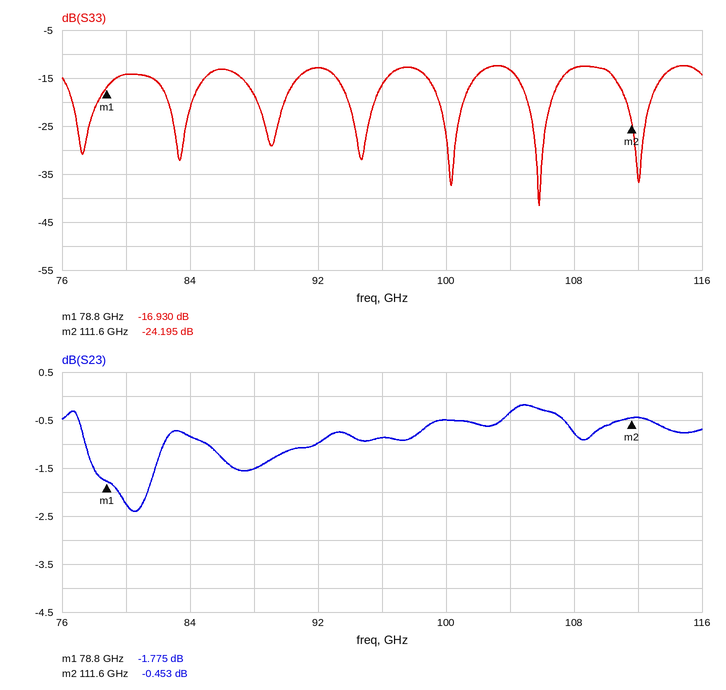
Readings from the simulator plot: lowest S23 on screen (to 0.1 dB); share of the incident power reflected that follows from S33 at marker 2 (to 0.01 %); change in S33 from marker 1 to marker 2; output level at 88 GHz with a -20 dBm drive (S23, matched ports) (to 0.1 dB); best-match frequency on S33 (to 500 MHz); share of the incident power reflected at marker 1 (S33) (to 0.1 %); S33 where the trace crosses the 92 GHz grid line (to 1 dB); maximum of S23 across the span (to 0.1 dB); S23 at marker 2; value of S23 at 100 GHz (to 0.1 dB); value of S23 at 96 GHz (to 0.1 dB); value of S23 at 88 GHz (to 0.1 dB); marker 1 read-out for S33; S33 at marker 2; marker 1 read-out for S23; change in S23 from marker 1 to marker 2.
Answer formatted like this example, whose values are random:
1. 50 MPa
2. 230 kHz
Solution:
1. -2.4 dB
2. 0.38 %
3. -7.265 dB
4. -21.5 dBm
5. 106.0 GHz
6. 2.0 %
7. -13 dB
8. -0.2 dB
9. -0.453 dB
10. -0.5 dB
11. -0.9 dB
12. -1.5 dB
13. -16.930 dB
14. -24.195 dB
15. -1.775 dB
16. 1.322 dB
